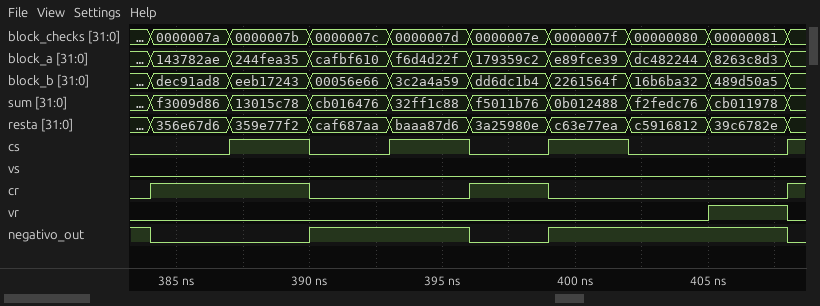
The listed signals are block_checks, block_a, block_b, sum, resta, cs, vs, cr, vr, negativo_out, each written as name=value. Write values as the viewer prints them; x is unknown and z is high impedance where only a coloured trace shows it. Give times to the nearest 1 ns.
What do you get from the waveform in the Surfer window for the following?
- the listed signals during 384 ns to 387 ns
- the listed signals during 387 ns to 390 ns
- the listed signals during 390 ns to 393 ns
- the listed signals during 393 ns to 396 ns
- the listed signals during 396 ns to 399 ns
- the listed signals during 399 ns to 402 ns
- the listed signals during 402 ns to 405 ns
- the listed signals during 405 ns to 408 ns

block_checks=0000007a, block_a=143782ae, block_b=dec91ad8, sum=f3009d86, resta=356e67d6, cs=0, vs=0, cr=1, vr=0, negativo_out=0
block_checks=0000007b, block_a=244fea35, block_b=eeb17243, sum=13015c78, resta=359e77f2, cs=1, vs=0, cr=1, vr=0, negativo_out=0
block_checks=0000007c, block_a=cafbf610, block_b=00056e66, sum=cb016476, resta=caf687aa, cs=0, vs=0, cr=0, vr=0, negativo_out=1
block_checks=0000007d, block_a=f6d4d22f, block_b=3c2a4a59, sum=32ff1c88, resta=baaa87d6, cs=1, vs=0, cr=0, vr=0, negativo_out=1
block_checks=0000007e, block_a=179359c2, block_b=dd6dc1b4, sum=f5011b76, resta=3a25980e, cs=0, vs=0, cr=1, vr=0, negativo_out=0
block_checks=0000007f, block_a=e89fce39, block_b=2261564f, sum=0b012488, resta=c63e77ea, cs=1, vs=0, cr=0, vr=0, negativo_out=1
block_checks=00000080, block_a=dc482244, block_b=16b6ba32, sum=f2fedc76, resta=c5916812, cs=0, vs=0, cr=0, vr=0, negativo_out=1
block_checks=00000081, block_a=8263c8d3, block_b=489d50a5, sum=cb011978, resta=39c6782e, cs=0, vs=0, cr=0, vr=1, negativo_out=1
